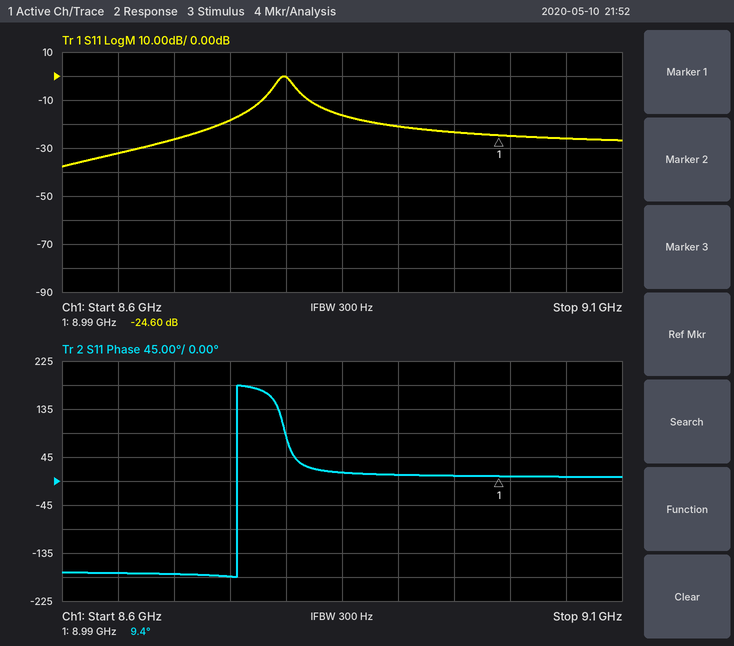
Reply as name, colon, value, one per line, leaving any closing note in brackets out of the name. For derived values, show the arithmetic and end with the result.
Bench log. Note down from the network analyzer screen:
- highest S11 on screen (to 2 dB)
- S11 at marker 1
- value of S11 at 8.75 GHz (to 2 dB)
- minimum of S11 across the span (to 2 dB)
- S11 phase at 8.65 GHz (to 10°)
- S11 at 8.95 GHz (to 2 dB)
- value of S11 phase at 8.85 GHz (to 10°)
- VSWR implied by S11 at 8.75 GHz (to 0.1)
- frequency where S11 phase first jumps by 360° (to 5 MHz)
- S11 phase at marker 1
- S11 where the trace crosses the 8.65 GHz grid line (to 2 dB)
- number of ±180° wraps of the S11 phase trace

highest S11 on screen: 0 dB
S11 at marker 1: -24.60 dB
value of S11 at 8.75 GHz: -18 dB
minimum of S11 across the span: -38 dB
S11 phase at 8.65 GHz: -170°
S11 at 8.95 GHz: -24 dB
value of S11 phase at 8.85 GHz: 20°
VSWR implied by S11 at 8.75 GHz: |Γ| = 10^(-18/20) = 0.1259; VSWR = (1 + 0.1259)/(1 − 0.1259) ≈ 1.3
frequency where S11 phase first jumps by 360°: 8.755 GHz
S11 phase at marker 1: 9.4°
S11 where the trace crosses the 8.65 GHz grid line: -32 dB
number of ±180° wraps of the S11 phase trace: 1
